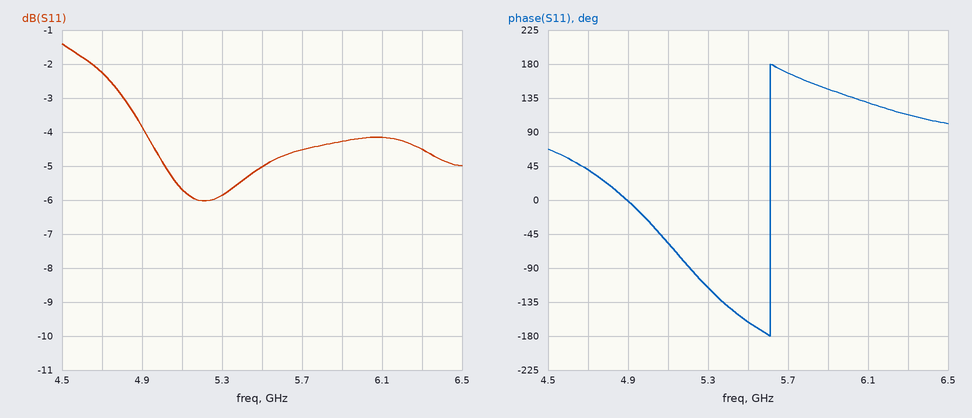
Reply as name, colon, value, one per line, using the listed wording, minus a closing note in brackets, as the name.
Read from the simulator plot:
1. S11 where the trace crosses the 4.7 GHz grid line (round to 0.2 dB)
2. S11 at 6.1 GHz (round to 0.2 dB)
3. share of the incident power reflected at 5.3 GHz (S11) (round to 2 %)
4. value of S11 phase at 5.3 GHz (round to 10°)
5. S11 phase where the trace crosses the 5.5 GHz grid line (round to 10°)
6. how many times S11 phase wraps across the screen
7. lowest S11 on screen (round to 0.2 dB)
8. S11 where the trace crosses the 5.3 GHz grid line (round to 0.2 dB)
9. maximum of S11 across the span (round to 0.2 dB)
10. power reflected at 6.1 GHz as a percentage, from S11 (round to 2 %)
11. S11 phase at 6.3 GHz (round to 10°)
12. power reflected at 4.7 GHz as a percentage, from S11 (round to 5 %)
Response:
S11 where the trace crosses the 4.7 GHz grid line: -2.2 dB
S11 at 6.1 GHz: -4.2 dB
share of the incident power reflected at 5.3 GHz (S11): 26 %
value of S11 phase at 5.3 GHz: -120°
S11 phase where the trace crosses the 5.5 GHz grid line: -160°
how many times S11 phase wraps across the screen: 1
lowest S11 on screen: -6.0 dB
S11 where the trace crosses the 5.3 GHz grid line: -5.8 dB
maximum of S11 across the span: -1.4 dB
power reflected at 6.1 GHz as a percentage, from S11: 38 %
S11 phase at 6.3 GHz: 110°
power reflected at 4.7 GHz as a percentage, from S11: 60 %
